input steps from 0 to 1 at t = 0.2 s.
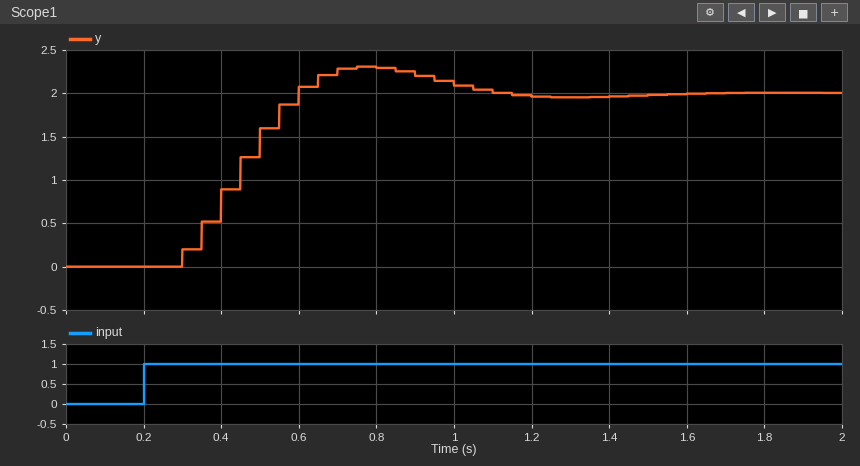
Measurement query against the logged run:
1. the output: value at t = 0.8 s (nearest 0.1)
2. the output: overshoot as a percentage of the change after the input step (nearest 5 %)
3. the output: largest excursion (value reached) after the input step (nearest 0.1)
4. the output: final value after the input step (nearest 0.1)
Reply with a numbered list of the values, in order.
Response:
1. 2.3
2. 15 %
3. 2.3
4. 2.0
